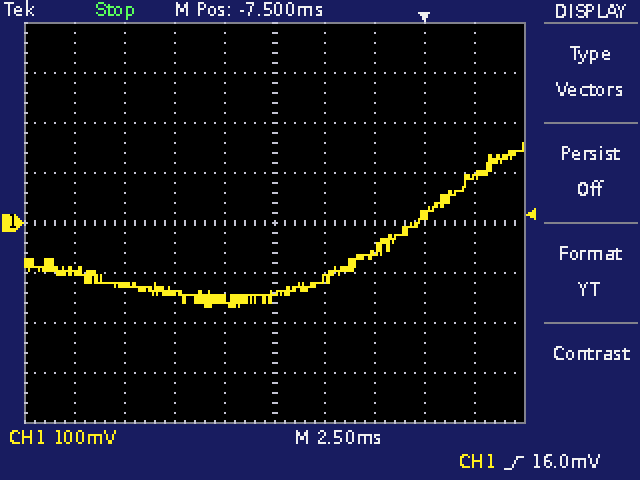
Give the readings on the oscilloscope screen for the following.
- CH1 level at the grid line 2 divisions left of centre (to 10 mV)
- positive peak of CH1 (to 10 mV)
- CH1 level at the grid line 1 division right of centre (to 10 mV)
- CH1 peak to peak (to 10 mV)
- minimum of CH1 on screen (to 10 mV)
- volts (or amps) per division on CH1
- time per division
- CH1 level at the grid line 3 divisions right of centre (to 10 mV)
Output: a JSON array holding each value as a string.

["-140 mV", "160 mV", "-110 mV", "330 mV", "-170 mV", "100 mV", "2.5 ms", "20 mV"]
